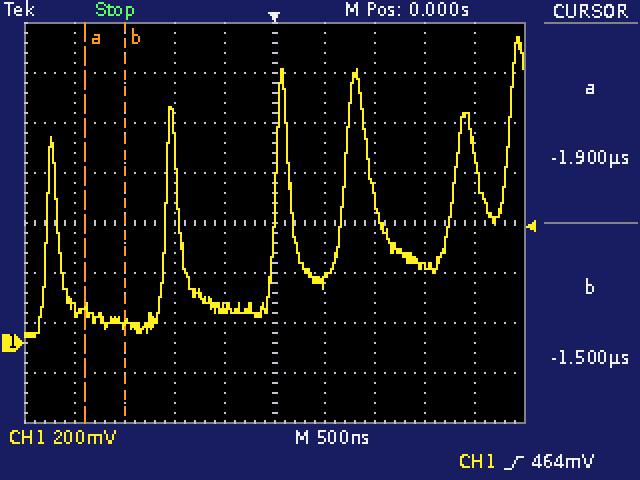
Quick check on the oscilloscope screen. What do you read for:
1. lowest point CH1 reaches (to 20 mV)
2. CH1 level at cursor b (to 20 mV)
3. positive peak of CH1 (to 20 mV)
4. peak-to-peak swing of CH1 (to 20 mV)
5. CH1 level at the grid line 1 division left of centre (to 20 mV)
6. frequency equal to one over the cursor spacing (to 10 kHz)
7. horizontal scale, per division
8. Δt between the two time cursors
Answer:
20 mV
80 mV
1.22 V
1.20 V
140 mV
2.50 MHz
500 ns
400 ns
